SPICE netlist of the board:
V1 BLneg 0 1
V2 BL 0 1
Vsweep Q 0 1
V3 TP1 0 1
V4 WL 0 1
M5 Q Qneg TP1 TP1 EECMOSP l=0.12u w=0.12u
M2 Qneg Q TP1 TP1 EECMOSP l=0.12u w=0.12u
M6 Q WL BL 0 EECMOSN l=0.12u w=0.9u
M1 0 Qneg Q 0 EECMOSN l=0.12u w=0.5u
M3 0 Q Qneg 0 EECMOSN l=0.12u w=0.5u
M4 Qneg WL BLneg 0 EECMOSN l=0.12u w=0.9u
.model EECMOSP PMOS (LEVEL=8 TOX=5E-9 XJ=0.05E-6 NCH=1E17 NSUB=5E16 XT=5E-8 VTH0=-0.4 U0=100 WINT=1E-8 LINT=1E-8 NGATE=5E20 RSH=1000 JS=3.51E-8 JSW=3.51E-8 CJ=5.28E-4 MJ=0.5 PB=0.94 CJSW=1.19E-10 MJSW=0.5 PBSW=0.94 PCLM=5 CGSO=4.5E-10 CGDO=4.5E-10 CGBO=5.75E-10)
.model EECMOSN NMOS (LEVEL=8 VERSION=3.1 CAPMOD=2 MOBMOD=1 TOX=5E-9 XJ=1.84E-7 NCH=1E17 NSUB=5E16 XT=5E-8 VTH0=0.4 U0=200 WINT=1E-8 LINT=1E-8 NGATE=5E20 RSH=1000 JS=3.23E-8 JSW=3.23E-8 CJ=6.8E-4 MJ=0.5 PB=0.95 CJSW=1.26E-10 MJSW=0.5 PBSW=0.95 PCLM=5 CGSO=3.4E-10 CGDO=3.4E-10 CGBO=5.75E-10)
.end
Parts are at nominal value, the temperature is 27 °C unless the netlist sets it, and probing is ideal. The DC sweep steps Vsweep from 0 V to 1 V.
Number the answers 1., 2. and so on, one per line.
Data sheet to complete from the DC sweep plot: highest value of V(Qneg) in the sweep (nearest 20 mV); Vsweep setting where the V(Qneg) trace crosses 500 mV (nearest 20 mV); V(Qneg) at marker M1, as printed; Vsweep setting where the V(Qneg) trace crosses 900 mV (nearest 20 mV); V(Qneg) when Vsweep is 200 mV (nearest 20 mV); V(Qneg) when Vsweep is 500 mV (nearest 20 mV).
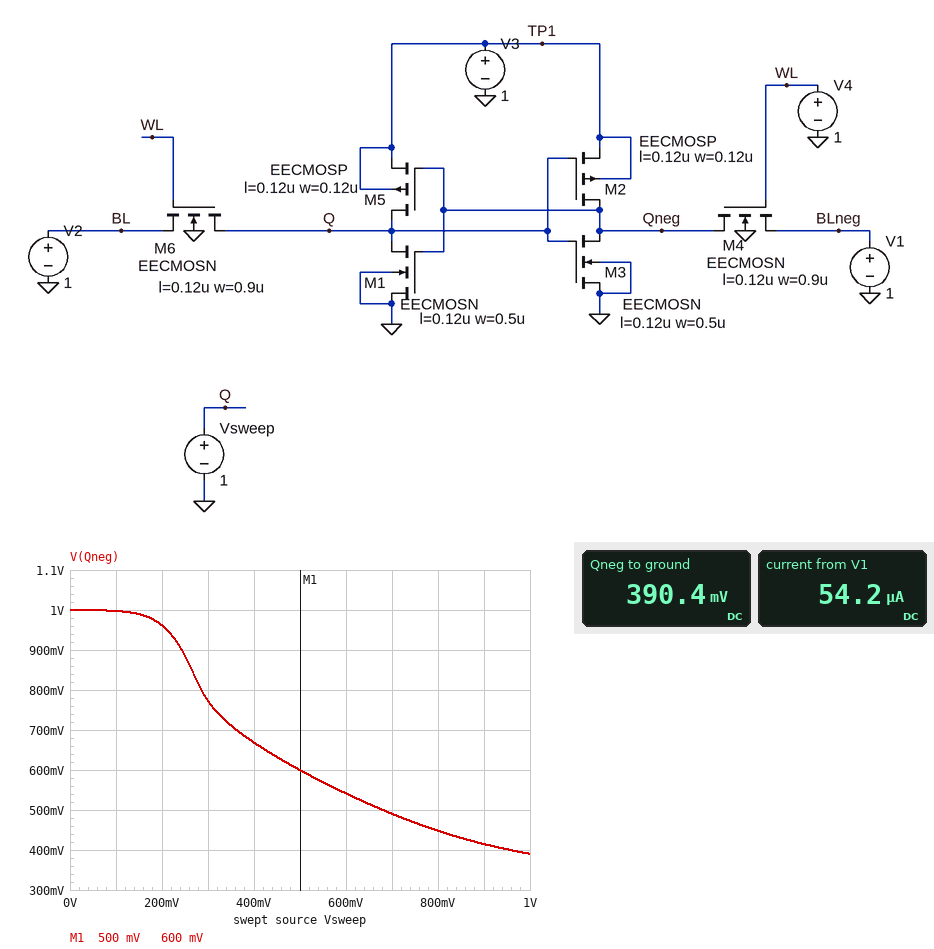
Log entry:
1. 1.00 V
2. 680 mV
3. 600 mV
4. 240 mV
5. 960 mV
6. 600 mV
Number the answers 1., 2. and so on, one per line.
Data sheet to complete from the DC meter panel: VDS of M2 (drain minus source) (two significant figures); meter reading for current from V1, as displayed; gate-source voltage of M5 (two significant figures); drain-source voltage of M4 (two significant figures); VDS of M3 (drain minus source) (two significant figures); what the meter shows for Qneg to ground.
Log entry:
1. -610 mV
2. 54.2 µA
3. -610 mV
4. -610 mV
5. -390 mV
6. 390.4 mV
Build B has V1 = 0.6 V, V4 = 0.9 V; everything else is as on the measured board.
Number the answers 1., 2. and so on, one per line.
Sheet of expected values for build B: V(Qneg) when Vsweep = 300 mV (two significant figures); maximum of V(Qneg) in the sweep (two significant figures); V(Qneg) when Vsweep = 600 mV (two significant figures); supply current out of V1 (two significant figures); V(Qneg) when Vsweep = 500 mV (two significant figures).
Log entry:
1. 630 mV
2. 840 mV
3. 390 mV
4. 42 µA
5. 450 mV
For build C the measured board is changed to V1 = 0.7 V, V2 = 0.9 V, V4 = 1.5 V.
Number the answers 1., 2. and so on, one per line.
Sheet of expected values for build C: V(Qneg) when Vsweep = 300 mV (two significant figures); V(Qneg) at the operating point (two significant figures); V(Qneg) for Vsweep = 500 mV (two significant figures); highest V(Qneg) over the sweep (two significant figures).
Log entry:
1. 700 mV
2. 450 mV
3. 630 mV
4. 730 mV
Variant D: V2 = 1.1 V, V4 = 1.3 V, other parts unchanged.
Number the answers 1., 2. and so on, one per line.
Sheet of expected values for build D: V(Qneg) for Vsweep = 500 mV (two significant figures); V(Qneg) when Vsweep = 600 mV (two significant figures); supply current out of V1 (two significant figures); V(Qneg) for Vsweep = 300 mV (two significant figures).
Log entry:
1. 800 mV
2. 740 mV
3. 66 µA
4. 940 mV
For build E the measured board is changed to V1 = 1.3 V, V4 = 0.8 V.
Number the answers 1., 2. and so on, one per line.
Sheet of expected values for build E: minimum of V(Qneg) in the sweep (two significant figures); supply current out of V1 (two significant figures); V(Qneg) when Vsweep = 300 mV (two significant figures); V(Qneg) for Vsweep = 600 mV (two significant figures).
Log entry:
1. 320 mV
2. 47 µA
3. 720 mV
4. 430 mV
